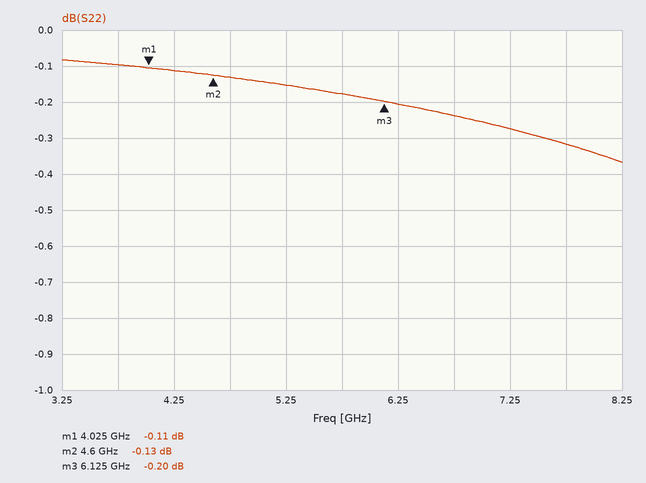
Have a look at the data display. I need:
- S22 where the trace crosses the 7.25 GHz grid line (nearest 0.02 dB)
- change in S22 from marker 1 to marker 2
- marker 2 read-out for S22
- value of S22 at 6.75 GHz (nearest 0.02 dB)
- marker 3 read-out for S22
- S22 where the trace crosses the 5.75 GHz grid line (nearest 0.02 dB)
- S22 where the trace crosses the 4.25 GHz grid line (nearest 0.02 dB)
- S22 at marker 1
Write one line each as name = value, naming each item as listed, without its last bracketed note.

S22 where the trace crosses the 7.25 GHz grid line = -0.28 dB
change in S22 from marker 1 to marker 2 = -0.02 dB
marker 2 read-out for S22 = -0.13 dB
value of S22 at 6.75 GHz = -0.24 dB
marker 3 read-out for S22 = -0.20 dB
S22 where the trace crosses the 5.75 GHz grid line = -0.18 dB
S22 where the trace crosses the 4.25 GHz grid line = -0.12 dB
S22 at marker 1 = -0.11 dB
